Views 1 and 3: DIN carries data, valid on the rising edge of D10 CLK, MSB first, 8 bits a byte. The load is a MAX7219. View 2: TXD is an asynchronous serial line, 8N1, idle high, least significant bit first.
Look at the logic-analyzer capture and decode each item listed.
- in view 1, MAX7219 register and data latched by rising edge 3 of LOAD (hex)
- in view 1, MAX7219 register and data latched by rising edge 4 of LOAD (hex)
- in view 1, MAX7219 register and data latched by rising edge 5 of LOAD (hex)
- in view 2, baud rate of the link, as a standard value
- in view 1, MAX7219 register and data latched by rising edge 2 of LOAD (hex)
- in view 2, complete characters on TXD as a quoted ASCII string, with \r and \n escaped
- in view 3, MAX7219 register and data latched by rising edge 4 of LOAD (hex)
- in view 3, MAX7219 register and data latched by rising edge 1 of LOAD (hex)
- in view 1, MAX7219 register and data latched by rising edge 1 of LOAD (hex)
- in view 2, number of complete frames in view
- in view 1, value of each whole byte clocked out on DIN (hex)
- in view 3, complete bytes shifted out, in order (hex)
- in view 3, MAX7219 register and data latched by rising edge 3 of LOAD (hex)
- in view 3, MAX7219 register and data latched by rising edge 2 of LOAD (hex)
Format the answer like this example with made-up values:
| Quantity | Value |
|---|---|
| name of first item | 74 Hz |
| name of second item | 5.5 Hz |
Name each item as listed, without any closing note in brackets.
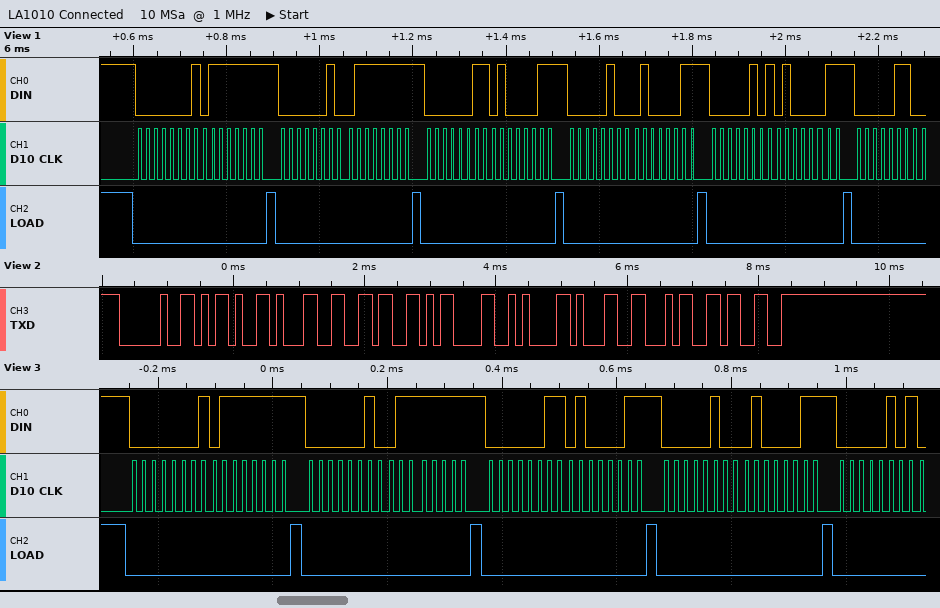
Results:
| Quantity | Value |
|---|---|
| in view 1, MAX7219 register and data latched by rising edge 3 of LOAD | register 0x3, data 0x43 |
| in view 1, MAX7219 register and data latched by rising edge 4 of LOAD | register 0x4, data 0x43 |
| in view 1, MAX7219 register and data latched by rising edge 5 of LOAD | register 0x5, data 0x43 |
| in view 2, baud rate of the link, as a standard value | 9600 baud |
| in view 1, MAX7219 register and data latched by rising edge 2 of LOAD | register 0x2, data 0x7F |
| in view 2, complete characters on TXD as a quoted ASCII string, with \r and \n escaped | " -16\r\n143" |
| in view 3, MAX7219 register and data latched by rising edge 4 of LOAD | register 0x4, data 0x43 |
| in view 3, MAX7219 register and data latched by rising edge 1 of LOAD | register 0x1, data 0x7F |
| in view 1, MAX7219 register and data latched by rising edge 1 of LOAD | register 0x1, data 0x7F |
| in view 2, number of complete frames in view | 9 |
| in view 1, value of each whole byte clocked out on DIN | 01 7F 02 7F 03 43 04 43 05 43 06 |
| in view 3, complete bytes shifted out, in order | 0x01 0x7F 0x02 0x7F 0x03 0x43 0x04 0x43 0x05 |
| in view 3, MAX7219 register and data latched by rising edge 3 of LOAD | register 0x3, data 0x43 |
| in view 3, MAX7219 register and data latched by rising edge 2 of LOAD | register 0x2, data 0x7F |
